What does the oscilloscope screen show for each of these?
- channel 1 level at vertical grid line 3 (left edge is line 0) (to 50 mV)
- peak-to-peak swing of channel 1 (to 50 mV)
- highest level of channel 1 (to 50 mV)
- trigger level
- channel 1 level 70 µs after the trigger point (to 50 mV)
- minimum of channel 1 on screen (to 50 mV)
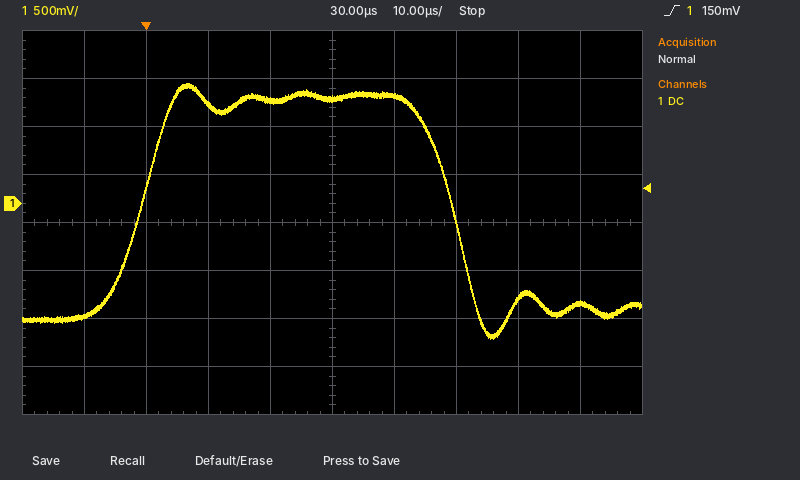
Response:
1.05 V
2.65 V
1.25 V
150 mV
-1.05 V
-1.40 V
